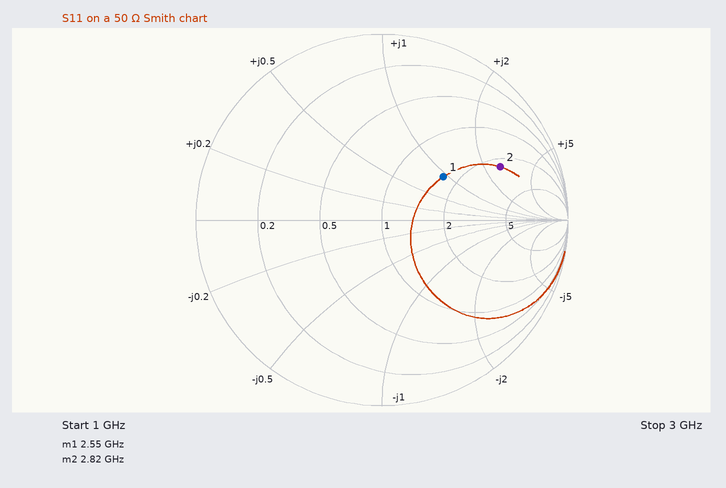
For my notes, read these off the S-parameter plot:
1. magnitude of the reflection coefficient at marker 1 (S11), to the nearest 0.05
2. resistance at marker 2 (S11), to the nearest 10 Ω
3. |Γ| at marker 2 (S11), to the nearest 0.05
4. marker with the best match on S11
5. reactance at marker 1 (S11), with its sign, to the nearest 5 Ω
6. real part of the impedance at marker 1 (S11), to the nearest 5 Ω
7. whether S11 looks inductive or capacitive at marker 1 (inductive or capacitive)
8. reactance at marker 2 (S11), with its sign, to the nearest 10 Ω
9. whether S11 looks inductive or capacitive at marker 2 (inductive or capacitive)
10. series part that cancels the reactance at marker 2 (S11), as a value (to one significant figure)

0.40
120 Ω
0.70
marker 1
+45 Ω
85 Ω
inductive
+130 Ω
inductive
400 fF
